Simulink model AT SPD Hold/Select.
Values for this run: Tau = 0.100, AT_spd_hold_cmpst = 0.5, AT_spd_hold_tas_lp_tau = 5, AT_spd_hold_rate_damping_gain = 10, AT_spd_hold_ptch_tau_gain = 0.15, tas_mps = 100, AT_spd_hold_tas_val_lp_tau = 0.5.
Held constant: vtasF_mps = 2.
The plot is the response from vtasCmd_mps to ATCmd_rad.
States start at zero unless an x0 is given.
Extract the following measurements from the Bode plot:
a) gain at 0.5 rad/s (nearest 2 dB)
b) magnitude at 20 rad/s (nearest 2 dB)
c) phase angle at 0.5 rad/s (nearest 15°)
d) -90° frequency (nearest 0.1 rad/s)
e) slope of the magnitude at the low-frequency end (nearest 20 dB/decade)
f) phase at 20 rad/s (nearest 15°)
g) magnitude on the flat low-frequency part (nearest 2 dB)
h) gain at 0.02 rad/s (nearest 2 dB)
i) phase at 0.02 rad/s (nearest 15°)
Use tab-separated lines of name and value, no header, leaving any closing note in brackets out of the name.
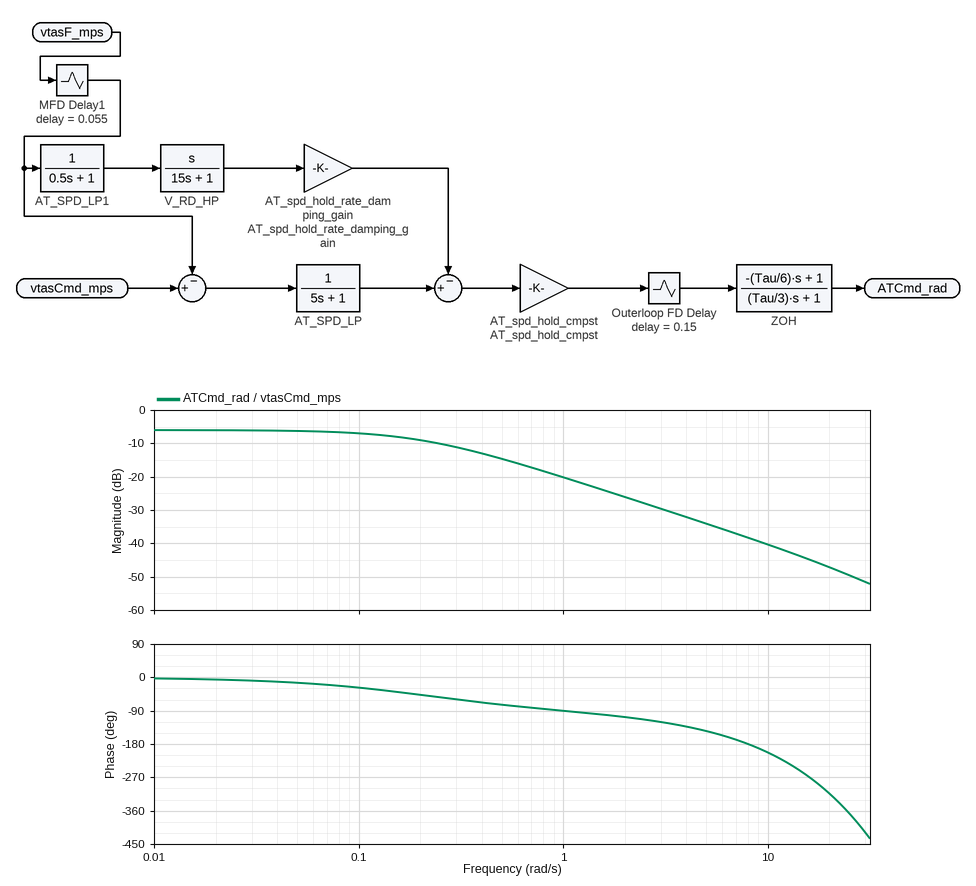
gain at 0.5 rad/s	-14 dB
magnitude at 20 rad/s	-48 dB
phase angle at 0.5 rad/s	-75°
-90° frequency	1.0 rad/s
slope of the magnitude at the low-frequency end	0 dB/decade
phase at 20 rad/s	-315°
magnitude on the flat low-frequency part	-6 dB
gain at 0.02 rad/s	-6 dB
phase at 0.02 rad/s	0°
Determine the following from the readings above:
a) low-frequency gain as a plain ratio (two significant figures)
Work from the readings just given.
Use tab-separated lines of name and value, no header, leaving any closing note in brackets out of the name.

low-frequency gain as a plain ratio	0.50
